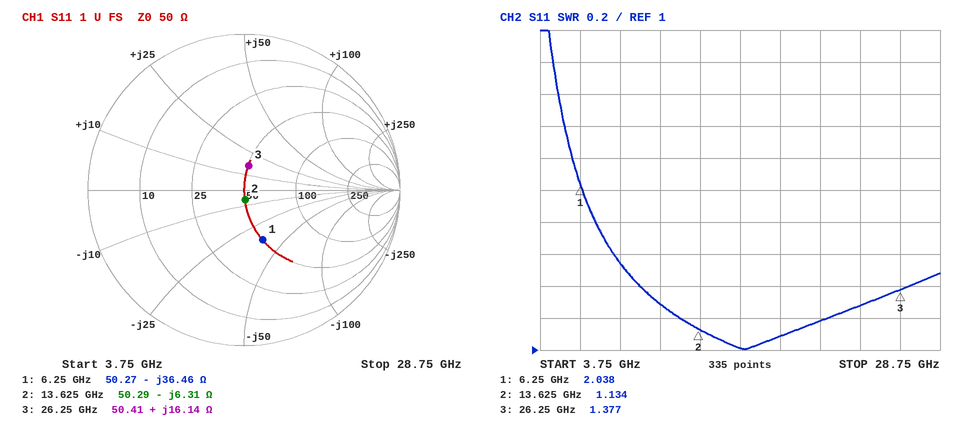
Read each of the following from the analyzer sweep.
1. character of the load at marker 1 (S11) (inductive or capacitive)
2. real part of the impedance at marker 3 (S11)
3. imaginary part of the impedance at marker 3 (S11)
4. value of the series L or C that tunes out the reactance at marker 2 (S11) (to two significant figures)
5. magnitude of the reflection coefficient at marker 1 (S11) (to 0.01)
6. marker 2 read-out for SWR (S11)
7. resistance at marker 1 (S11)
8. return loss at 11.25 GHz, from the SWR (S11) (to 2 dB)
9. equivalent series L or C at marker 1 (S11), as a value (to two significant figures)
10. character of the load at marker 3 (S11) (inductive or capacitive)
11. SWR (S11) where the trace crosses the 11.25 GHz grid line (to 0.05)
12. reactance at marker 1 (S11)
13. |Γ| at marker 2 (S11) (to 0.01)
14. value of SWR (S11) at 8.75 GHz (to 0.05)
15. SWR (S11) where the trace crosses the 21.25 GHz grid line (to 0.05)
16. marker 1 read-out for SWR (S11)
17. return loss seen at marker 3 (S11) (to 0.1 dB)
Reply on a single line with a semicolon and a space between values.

capacitive; 50.41 Ω; +16.14 Ω; 74 pH; 0.34; 1.134; 50.27 Ω; 18 dB; 700 fF; inductive; 1.30; -36.46 Ω; 0.06; 1.55; 1.20; 2.038; 16.0 dB
